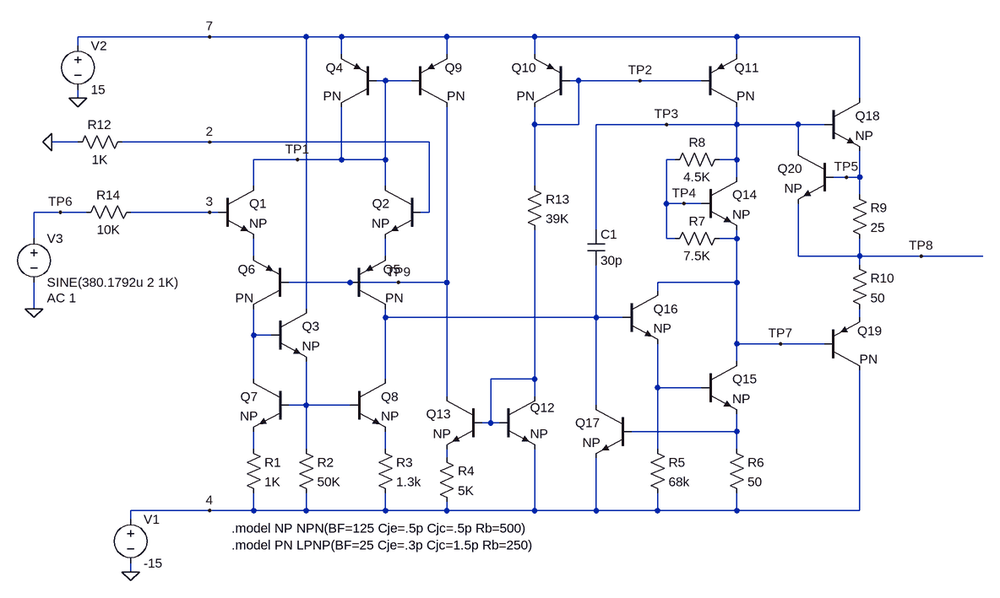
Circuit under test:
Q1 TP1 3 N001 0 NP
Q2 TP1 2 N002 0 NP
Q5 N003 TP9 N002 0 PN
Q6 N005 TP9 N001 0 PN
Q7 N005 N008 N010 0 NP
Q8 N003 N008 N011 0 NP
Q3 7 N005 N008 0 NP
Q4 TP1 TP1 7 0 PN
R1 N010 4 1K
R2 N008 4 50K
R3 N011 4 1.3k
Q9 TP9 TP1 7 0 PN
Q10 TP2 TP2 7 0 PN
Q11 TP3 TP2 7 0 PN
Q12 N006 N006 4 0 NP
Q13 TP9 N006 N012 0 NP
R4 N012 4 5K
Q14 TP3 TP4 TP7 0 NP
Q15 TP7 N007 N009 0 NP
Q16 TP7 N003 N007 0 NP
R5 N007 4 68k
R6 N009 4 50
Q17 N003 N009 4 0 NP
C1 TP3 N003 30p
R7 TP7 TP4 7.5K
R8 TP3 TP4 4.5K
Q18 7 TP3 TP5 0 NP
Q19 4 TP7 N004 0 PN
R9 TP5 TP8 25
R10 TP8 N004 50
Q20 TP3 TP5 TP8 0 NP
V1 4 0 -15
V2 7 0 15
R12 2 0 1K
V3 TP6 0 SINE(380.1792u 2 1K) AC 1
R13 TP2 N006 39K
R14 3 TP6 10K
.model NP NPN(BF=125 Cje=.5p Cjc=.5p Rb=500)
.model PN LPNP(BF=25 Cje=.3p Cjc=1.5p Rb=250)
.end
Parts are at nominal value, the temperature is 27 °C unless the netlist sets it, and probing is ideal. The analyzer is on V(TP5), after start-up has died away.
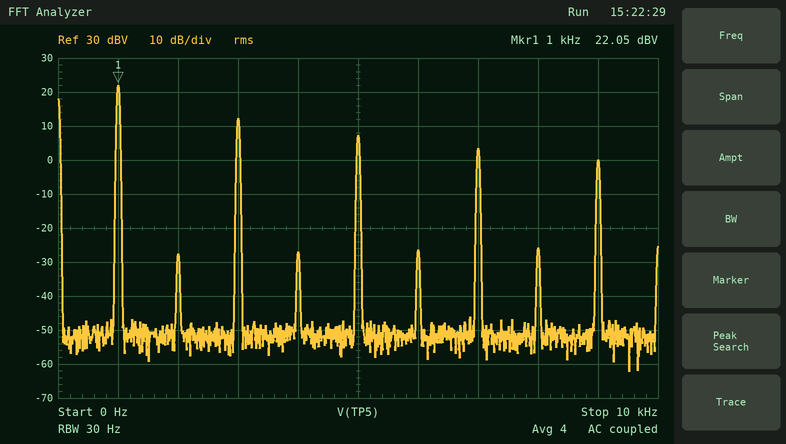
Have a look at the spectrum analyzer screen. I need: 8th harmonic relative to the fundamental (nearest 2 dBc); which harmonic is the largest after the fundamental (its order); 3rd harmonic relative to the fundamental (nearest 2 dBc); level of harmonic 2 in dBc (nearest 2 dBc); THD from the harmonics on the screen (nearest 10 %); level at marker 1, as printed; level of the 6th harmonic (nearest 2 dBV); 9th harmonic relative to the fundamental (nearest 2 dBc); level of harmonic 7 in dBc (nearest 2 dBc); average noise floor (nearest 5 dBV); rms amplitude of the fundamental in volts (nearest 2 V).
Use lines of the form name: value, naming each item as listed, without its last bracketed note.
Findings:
8th harmonic relative to the fundamental: -48 dBc
which harmonic is the largest after the fundamental: 3
3rd harmonic relative to the fundamental: -10 dBc
level of harmonic 2 in dBc: -50 dBc
THD from the harmonics on the screen: 40 %
level at marker 1, as printed: 22.05 dBV
level of the 6th harmonic: -26 dBV
9th harmonic relative to the fundamental: -22 dBc
level of harmonic 7 in dBc: -18 dBc
average noise floor: -50 dBV
rms amplitude of the fundamental in volts: 12 V
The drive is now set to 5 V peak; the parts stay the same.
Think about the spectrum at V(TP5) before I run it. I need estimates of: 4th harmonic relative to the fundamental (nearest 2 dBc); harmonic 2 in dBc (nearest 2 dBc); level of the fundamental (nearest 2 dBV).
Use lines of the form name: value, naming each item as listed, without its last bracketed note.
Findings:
4th harmonic relative to the fundamental: -52 dBc
harmonic 2 in dBc: -52 dBc
level of the fundamental: 22 dBV
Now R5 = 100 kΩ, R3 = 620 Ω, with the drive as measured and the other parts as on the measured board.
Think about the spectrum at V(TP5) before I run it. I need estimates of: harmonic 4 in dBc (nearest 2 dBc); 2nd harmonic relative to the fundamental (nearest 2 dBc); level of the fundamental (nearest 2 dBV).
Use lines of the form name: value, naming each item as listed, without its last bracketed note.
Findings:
harmonic 4 in dBc: -34 dBc
2nd harmonic relative to the fundamental: -34 dBc
level of the fundamental: 22 dBV
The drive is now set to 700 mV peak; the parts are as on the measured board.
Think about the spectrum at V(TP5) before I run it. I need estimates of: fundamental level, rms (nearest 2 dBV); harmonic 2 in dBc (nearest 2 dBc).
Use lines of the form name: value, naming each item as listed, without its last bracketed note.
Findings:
fundamental level, rms: 22 dBV
harmonic 2 in dBc: -46 dBc
